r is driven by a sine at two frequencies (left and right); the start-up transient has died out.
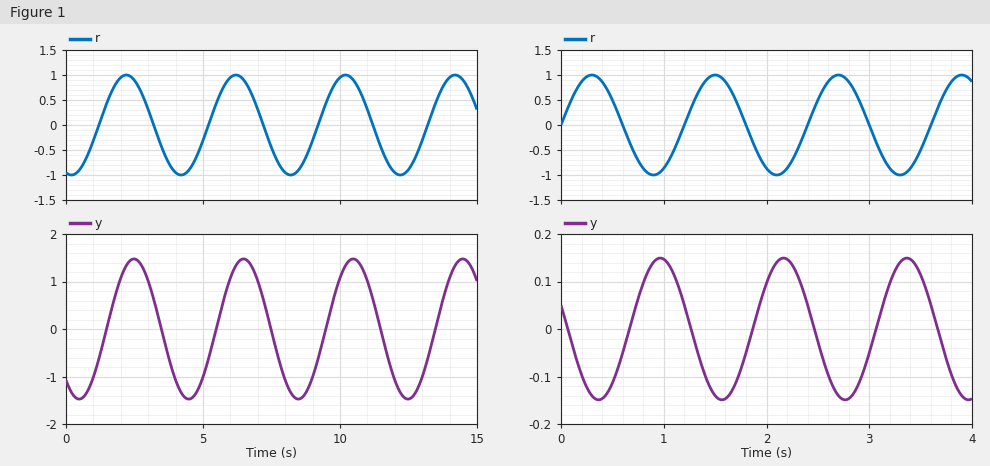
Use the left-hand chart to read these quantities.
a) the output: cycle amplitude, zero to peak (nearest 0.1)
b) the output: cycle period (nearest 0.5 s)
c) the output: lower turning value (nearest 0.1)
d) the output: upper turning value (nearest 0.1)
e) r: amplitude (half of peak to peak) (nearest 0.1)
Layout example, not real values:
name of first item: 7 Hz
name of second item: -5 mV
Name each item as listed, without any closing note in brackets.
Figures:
the output: cycle amplitude, zero to peak: 1.5
the output: cycle period: 4.0 s
the output: lower turning value: -1.5
the output: upper turning value: 1.5
r: amplitude (half of peak to peak): 1.0
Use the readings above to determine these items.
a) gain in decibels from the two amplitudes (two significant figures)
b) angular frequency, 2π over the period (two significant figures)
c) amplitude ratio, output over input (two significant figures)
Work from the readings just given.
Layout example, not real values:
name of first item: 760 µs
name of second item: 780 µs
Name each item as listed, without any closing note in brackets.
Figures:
gain in decibels from the two amplitudes: 3.5 dB
angular frequency, 2π over the period: 1.6 rad/s
amplitude ratio, output over input: 1.5
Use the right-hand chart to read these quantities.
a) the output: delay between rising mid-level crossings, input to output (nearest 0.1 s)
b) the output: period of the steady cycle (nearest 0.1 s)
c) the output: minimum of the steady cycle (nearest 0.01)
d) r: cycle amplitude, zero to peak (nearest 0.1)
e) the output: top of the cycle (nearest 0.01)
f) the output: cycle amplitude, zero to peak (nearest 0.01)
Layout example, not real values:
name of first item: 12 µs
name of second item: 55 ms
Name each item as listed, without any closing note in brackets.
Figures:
the output: delay between rising mid-level crossings, input to output: 0.7 s
the output: period of the steady cycle: 1.2 s
the output: minimum of the steady cycle: -0.15
r: cycle amplitude, zero to peak: 1.0
the output: top of the cycle: 0.15
the output: cycle amplitude, zero to peak: 0.15
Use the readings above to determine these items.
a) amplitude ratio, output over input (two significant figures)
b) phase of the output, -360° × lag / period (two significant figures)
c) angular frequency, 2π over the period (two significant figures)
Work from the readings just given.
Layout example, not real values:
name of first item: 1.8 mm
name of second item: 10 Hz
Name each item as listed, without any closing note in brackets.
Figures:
amplitude ratio, output over input: 0.15
phase of the output, -360° × lag / period: -210°
angular frequency, 2π over the period: 5.2 rad/s
